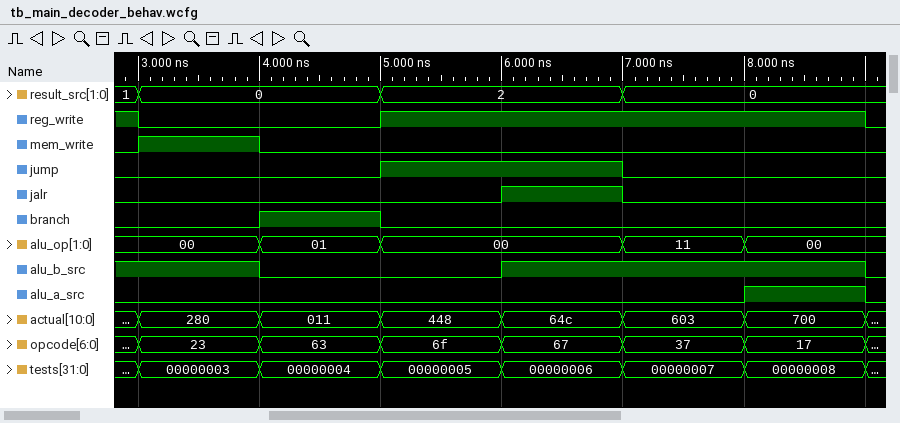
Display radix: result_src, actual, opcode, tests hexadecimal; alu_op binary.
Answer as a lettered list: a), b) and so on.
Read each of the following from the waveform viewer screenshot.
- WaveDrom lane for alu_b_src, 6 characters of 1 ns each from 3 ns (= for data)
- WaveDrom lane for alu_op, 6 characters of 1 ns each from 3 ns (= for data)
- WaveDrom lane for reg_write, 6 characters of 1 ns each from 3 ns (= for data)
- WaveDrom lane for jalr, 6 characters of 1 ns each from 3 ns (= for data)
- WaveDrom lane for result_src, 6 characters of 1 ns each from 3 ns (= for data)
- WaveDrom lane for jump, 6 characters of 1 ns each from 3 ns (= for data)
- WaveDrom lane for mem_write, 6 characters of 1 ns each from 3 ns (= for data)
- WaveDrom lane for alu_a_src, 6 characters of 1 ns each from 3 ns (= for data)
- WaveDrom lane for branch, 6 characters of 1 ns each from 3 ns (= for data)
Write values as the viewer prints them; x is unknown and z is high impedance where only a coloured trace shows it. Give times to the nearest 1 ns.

a) {name: 'alu_b_src', wave: '10.1..'}
b) {name: 'alu_op', wave: '===.==', data: '00 01 00 11 00'}
c) {name: 'reg_write', wave: '0.1...'}
d) {name: 'jalr', wave: '0..10.'}
e) {name: 'result_src', wave: '=.=.=.', data: '0 2 0'}
f) {name: 'jump', wave: '0.1.0.'}
g) {name: 'mem_write', wave: '10....'}
h) {name: 'alu_a_src', wave: '0....1'}
i) {name: 'branch', wave: '010...'}
